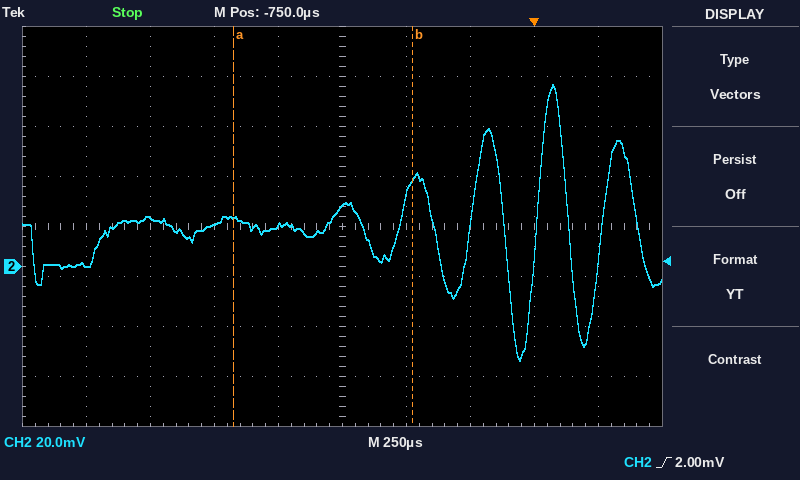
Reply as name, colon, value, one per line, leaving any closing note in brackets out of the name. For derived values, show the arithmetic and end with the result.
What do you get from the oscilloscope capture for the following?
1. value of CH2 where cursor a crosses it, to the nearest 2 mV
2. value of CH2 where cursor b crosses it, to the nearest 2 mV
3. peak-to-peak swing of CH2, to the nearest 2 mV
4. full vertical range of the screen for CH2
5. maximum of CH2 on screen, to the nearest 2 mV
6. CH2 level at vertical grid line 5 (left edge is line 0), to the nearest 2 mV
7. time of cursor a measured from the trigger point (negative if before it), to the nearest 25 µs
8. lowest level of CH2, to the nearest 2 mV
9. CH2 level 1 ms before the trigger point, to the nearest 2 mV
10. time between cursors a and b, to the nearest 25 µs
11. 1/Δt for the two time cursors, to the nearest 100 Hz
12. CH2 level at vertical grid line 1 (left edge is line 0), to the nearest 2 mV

value of CH2 where cursor a crosses it, to the nearest 2 mV: 20 mV
value of CH2 where cursor b crosses it, to the nearest 2 mV: 34 mV
peak-to-peak swing of CH2, to the nearest 2 mV: 72 mV − (-38 mV) = 110 mV
full vertical range of the screen for CH2: 160 mV
maximum of CH2 on screen, to the nearest 2 mV: 72 mV
CH2 level at vertical grid line 5 (left edge is line 0), to the nearest 2 mV: 24 mV
time of cursor a measured from the trigger point (negative if before it), to the nearest 25 µs: -1.175 ms
lowest level of CH2, to the nearest 2 mV: -38 mV
CH2 level 1 ms before the trigger point, to the nearest 2 mV: 16 mV
time between cursors a and b, to the nearest 25 µs: 700 µs
1/Δt for the two time cursors, to the nearest 100 Hz: 1 / 700 µs ≈ 1.4 kHz
CH2 level at vertical grid line 1 (left edge is line 0), to the nearest 2 mV: 0 mV
